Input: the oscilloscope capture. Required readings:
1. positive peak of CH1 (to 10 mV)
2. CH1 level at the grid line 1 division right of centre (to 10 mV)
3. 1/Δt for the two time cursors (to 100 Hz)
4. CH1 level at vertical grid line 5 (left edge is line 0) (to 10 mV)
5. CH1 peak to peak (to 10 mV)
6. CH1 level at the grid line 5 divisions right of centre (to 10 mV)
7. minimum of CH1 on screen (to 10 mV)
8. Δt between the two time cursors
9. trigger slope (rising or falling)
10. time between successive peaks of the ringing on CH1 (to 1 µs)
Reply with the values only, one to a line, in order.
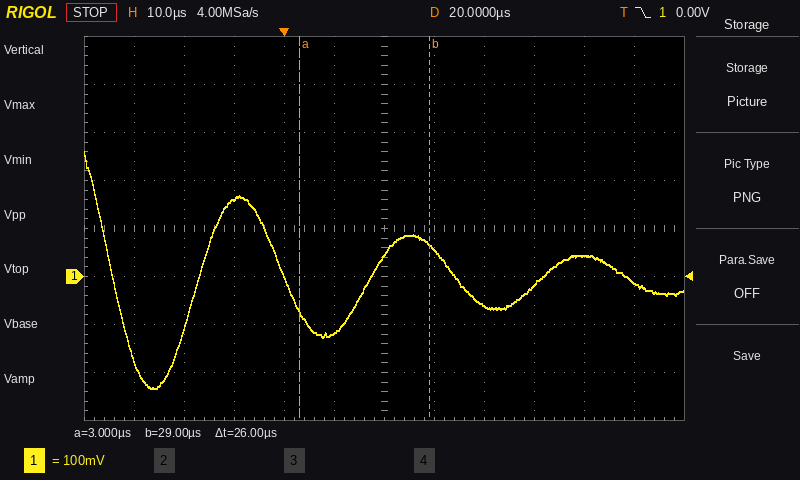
260 mV
60 mV
38.5 kHz
-120 mV
490 mV
-10 mV
-230 mV
26 µs
falling
34 µs
